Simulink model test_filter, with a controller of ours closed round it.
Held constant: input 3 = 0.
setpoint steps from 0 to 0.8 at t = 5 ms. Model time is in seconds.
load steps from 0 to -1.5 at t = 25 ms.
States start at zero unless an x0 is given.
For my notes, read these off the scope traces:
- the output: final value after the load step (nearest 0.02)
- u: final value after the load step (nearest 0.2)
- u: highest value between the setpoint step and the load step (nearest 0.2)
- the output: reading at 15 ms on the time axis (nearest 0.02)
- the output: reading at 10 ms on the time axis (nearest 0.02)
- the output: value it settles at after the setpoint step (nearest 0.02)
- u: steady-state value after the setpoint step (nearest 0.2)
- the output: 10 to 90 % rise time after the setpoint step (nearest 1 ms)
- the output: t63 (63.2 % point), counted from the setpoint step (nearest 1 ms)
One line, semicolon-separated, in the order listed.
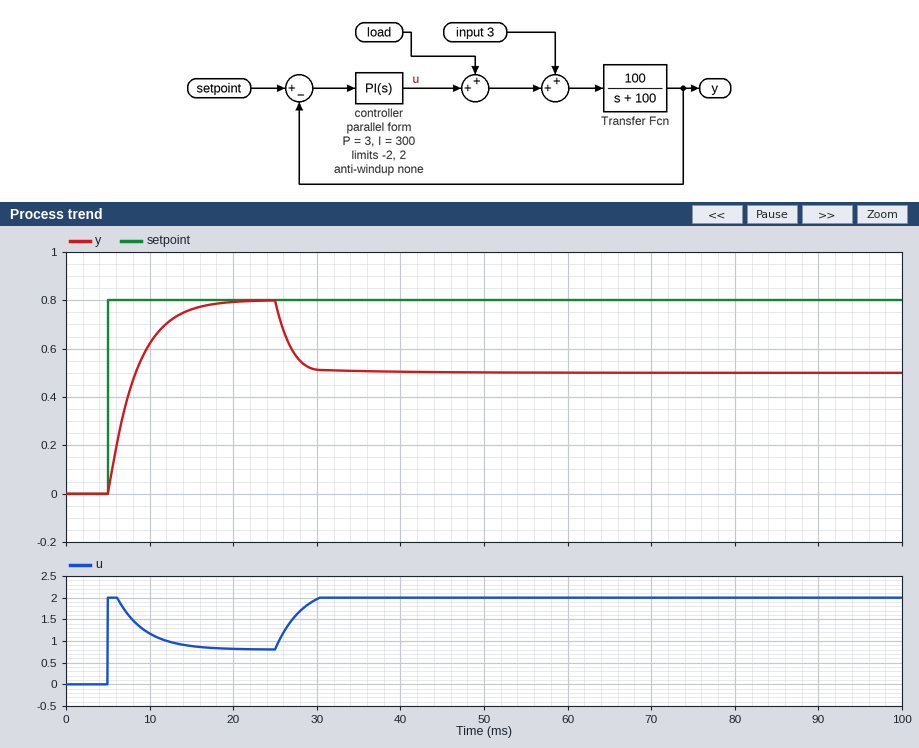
0.50; 2.0; 2.0; 0.76; 0.62; 0.80; 0.8; 7 ms; 3 ms
